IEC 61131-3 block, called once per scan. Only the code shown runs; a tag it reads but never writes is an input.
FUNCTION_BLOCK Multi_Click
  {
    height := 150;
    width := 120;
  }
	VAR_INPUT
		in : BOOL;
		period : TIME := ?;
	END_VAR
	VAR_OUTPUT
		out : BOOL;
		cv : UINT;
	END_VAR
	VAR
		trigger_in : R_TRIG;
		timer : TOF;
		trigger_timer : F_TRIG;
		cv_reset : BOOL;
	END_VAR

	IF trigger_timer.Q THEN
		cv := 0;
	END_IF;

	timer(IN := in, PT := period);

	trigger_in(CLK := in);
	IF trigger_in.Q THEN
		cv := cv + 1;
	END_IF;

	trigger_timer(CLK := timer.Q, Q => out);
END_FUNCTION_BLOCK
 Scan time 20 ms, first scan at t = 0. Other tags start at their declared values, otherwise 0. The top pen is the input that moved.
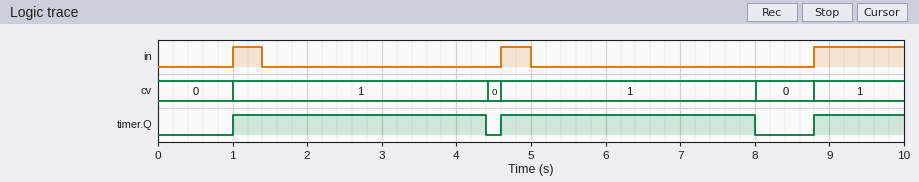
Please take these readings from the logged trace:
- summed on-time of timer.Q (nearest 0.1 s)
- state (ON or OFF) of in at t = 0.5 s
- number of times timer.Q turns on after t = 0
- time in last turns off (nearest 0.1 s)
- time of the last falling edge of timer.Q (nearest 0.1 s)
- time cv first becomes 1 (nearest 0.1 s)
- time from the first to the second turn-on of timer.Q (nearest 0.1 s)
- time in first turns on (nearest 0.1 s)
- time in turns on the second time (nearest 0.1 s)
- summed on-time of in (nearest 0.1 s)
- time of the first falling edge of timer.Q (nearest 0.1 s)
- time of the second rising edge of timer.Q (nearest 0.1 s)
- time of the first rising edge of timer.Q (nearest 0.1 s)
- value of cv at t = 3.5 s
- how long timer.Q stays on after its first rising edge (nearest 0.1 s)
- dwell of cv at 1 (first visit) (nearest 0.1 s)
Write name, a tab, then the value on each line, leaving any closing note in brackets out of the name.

summed on-time of timer.Q	8.0 s
state (ON or OFF) of in at t = 0.5 s	OFF
number of times timer.Q turns on after t = 0	3
time in last turns off	5.0 s
time of the last falling edge of timer.Q	8.0 s
time cv first becomes 1	1.0 s
time from the first to the second turn-on of timer.Q	3.6 s
time in first turns on	1.0 s
time in turns on the second time	4.6 s
summed on-time of in	2.0 s
time of the first falling edge of timer.Q	4.4 s
time of the second rising edge of timer.Q	4.6 s
time of the first rising edge of timer.Q	1.0 s
value of cv at t = 3.5 s	1
how long timer.Q stays on after its first rising edge	3.4 s
dwell of cv at 1 (first visit)	3.4 s
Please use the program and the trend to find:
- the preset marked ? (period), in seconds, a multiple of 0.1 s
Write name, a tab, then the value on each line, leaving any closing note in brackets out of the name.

the preset marked ? (period), in seconds, a multiple of 0.1 s	3.0 s
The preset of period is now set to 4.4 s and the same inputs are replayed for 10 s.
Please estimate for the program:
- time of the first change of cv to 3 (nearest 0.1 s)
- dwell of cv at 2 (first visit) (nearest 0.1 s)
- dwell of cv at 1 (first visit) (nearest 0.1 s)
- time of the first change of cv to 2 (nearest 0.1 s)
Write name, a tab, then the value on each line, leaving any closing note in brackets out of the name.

time of the first change of cv to 3	8.8 s
dwell of cv at 2 (first visit)	4.2 s
dwell of cv at 1 (first visit)	3.6 s
time of the first change of cv to 2	4.6 s
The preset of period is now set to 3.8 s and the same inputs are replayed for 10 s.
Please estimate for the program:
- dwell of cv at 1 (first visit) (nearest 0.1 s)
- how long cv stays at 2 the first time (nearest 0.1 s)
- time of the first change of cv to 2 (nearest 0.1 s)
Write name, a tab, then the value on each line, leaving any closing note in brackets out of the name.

dwell of cv at 1 (first visit)	3.6 s
how long cv stays at 2 the first time	4.2 s
time of the first change of cv to 2	4.6 s
